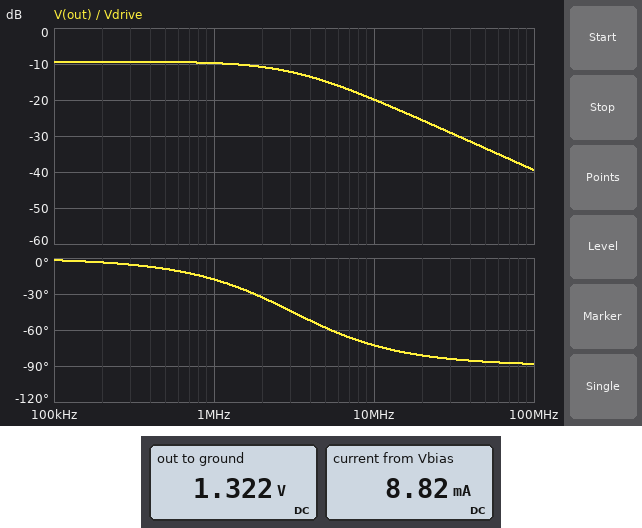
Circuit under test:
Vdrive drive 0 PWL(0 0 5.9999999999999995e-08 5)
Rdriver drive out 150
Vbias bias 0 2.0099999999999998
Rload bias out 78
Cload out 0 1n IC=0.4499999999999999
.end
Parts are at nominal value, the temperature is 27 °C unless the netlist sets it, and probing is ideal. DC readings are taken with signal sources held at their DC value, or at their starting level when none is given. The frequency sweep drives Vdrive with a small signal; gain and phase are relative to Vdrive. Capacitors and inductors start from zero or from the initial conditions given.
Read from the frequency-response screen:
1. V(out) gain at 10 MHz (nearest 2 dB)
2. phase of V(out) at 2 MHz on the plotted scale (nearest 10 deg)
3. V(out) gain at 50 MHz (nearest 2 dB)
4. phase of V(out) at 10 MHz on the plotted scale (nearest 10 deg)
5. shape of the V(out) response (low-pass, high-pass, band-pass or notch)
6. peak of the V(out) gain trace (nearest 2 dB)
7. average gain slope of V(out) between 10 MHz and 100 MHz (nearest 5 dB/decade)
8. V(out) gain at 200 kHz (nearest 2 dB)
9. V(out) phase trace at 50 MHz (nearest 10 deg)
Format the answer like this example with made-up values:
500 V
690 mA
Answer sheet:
-20 dB
-30 deg
-34 dB
-70 deg
low-pass
-10 dB
-20 dB/decade
-10 dB
-90 deg
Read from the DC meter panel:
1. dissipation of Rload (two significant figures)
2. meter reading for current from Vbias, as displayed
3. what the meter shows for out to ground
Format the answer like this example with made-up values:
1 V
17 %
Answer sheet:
6.1 mW
8.82 mA
1.322 V
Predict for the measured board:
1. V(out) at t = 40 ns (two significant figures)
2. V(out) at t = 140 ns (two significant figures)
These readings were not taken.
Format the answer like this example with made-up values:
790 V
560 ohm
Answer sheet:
1.3 V
2.8 V
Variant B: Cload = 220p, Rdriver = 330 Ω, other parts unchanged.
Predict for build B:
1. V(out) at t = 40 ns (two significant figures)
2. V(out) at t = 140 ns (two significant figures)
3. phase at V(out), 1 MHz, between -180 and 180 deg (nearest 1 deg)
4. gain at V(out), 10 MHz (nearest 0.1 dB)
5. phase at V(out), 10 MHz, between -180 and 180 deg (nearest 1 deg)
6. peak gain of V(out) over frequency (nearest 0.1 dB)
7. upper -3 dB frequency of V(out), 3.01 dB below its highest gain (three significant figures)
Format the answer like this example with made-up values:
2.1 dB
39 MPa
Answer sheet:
2.0 V
2.6 V
-5 deg
-16.8 dB
-41 deg
-14.4 dB
11.5 MHz
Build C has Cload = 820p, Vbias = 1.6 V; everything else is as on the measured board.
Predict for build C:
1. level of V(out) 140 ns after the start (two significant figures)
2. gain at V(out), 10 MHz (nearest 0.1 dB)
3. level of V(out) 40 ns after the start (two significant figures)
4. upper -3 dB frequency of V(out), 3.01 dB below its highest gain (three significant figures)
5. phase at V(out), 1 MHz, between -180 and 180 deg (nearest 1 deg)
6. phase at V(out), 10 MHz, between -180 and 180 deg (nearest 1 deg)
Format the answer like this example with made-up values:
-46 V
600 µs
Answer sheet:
2.6 V
-18.3 dB
1.2 V
3.78 MHz
-15 deg
-69 deg
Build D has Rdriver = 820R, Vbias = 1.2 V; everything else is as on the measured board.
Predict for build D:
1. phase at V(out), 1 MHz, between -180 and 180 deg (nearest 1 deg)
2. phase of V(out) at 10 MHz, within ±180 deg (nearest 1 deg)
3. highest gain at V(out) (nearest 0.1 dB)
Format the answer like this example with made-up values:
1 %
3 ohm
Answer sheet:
-24 deg
-77 deg
-21.2 dB
